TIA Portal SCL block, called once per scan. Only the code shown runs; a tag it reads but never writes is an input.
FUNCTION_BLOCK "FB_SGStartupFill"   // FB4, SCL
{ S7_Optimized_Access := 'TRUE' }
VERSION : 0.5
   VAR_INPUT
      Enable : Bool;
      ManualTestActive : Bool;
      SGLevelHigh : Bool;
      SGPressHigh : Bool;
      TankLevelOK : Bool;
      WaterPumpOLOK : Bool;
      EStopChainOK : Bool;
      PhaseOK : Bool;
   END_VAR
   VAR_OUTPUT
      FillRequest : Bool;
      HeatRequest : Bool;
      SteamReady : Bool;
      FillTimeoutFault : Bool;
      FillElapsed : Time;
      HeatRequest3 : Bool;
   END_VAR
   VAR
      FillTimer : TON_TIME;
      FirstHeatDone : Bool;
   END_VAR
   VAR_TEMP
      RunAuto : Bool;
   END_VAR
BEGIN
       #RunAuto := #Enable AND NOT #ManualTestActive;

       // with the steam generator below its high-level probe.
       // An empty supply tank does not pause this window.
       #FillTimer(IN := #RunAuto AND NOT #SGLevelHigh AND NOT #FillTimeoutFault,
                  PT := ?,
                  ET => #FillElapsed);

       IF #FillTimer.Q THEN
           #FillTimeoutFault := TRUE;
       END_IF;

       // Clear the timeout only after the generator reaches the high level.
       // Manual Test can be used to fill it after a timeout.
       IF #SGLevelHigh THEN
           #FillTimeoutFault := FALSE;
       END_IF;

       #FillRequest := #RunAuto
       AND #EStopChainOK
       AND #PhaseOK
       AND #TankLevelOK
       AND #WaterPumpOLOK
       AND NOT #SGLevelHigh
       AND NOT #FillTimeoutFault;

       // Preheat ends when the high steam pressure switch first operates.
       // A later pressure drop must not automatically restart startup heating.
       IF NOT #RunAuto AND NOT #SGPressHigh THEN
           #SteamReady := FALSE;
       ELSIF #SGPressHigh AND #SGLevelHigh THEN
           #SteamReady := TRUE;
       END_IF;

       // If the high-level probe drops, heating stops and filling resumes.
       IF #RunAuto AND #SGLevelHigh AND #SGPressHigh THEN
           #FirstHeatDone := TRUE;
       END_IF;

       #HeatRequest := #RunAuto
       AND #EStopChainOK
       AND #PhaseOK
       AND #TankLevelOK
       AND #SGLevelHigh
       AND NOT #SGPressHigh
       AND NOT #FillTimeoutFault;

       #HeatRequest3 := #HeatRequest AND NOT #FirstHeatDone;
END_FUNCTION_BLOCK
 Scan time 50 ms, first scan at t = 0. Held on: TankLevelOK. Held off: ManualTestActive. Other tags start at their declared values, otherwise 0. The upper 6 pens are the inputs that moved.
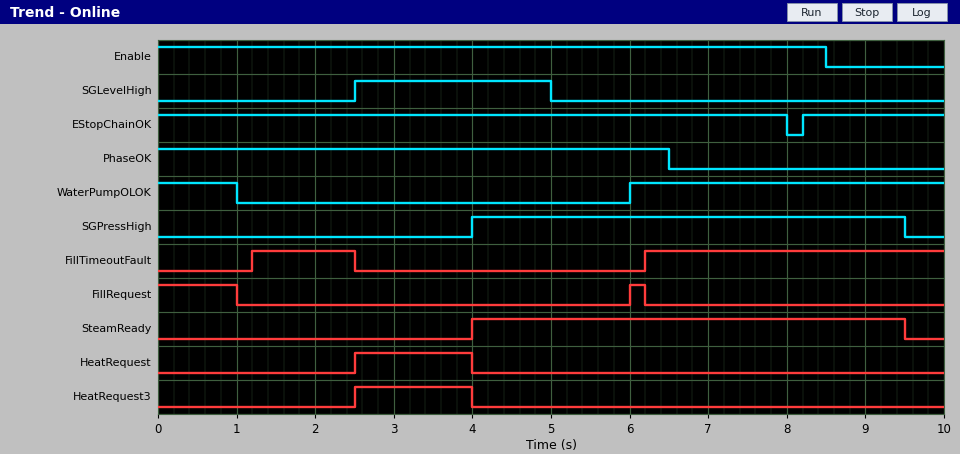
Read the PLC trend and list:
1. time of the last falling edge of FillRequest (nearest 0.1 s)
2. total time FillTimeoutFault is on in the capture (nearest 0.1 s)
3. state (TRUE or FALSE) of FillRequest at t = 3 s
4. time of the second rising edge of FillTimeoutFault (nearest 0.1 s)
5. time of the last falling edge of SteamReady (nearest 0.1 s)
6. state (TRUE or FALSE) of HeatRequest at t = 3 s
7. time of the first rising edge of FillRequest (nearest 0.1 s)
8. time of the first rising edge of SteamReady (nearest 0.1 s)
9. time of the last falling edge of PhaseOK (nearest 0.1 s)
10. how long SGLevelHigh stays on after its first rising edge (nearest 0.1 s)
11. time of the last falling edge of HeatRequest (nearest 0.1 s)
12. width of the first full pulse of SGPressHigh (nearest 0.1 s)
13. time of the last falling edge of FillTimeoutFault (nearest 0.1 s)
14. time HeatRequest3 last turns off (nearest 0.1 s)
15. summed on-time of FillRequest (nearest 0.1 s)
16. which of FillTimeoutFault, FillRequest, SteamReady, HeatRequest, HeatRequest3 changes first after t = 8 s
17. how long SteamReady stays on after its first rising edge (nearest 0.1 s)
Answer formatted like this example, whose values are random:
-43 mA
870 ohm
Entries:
6.2 s
5.1 s
FALSE
6.2 s
9.5 s
TRUE
6.0 s
4.0 s
6.5 s
2.5 s
4.0 s
5.5 s
2.5 s
4.0 s
1.2 s
SteamReady
5.5 s
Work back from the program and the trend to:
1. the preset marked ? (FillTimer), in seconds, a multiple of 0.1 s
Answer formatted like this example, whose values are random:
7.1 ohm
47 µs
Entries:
1.2 s
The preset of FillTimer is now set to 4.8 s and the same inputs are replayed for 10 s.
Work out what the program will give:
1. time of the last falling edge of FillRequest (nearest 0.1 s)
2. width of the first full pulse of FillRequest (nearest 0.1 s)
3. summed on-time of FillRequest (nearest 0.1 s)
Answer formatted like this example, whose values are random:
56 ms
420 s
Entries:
6.5 s
0.5 s
1.5 s
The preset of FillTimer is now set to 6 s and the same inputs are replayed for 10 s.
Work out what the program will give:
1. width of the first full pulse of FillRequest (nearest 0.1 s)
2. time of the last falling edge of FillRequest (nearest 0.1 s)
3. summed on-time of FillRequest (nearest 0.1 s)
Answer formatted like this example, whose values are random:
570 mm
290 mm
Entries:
0.5 s
6.5 s
1.5 s
